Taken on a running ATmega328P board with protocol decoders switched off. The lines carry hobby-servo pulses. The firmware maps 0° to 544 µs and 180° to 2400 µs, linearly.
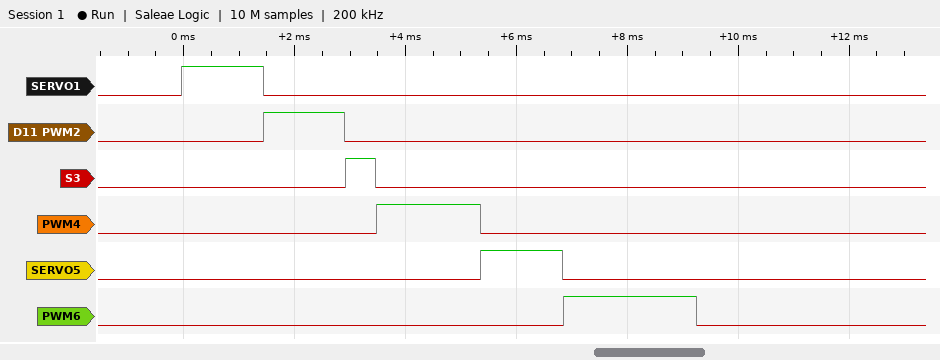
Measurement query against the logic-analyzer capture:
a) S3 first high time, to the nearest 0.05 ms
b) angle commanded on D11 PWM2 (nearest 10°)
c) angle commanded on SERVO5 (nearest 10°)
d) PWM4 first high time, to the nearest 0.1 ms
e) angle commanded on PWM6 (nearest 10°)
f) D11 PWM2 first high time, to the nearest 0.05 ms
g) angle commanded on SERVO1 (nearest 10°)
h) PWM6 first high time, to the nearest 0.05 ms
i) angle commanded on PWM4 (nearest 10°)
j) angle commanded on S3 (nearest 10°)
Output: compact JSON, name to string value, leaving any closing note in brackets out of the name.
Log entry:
{"S3 first high time, to the nearest 0.05 ms": "0.55 ms", "angle commanded on D11 PWM2": "90°", "angle commanded on SERVO5": "90°", "PWM4 first high time, to the nearest 0.1 ms": "1.9 ms", "angle commanded on PWM6": "180°", "D11 PWM2 first high time, to the nearest 0.05 ms": "1.45 ms", "angle commanded on SERVO1": "90°", "PWM6 first high time, to the nearest 0.05 ms": "2.40 ms", "angle commanded on PWM4": "130°", "angle commanded on S3": "0°"}
